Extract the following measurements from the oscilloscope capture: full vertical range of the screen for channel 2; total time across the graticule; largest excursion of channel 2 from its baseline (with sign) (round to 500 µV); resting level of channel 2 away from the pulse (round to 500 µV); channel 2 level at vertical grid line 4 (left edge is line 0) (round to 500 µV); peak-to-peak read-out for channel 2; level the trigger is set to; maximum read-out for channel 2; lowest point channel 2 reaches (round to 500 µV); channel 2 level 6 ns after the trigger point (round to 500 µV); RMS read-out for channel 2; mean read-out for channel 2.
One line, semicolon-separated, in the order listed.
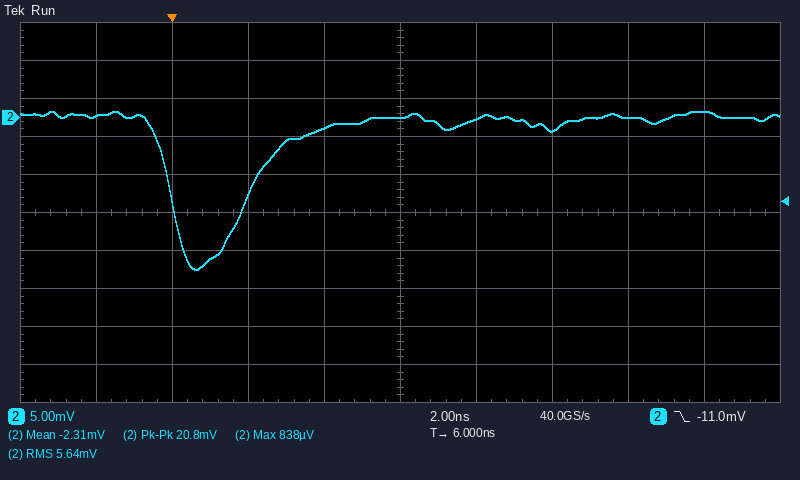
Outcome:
50 mV; 20 ns; -20.0 mV; 0.0 mV; -1.5 mV; 20.8 mV; -11.0 mV; 838 µV; -20.0 mV; 0.0 mV; 5.64 mV; -2.31 mV
